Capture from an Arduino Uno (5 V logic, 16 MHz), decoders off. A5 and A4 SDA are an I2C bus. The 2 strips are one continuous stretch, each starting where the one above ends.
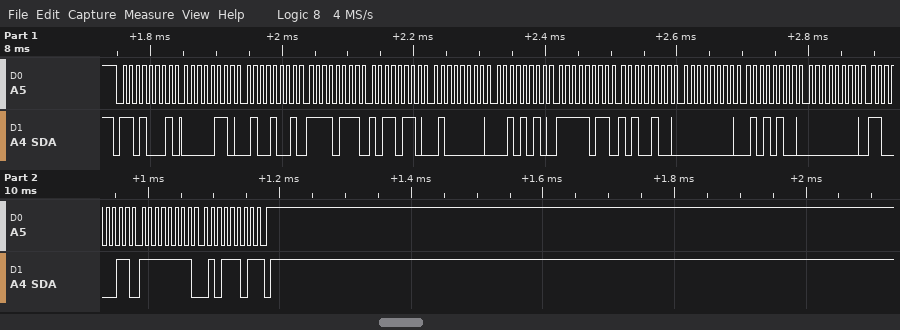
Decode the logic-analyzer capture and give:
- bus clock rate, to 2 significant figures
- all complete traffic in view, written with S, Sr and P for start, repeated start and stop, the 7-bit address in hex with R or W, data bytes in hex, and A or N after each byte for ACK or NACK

100 kHz
S 68R A 06 A 49 A F7 A B6 A 40 A 2A A FB A A4 A 00 A 54 A 00 A C3 A FF A 5D N P
